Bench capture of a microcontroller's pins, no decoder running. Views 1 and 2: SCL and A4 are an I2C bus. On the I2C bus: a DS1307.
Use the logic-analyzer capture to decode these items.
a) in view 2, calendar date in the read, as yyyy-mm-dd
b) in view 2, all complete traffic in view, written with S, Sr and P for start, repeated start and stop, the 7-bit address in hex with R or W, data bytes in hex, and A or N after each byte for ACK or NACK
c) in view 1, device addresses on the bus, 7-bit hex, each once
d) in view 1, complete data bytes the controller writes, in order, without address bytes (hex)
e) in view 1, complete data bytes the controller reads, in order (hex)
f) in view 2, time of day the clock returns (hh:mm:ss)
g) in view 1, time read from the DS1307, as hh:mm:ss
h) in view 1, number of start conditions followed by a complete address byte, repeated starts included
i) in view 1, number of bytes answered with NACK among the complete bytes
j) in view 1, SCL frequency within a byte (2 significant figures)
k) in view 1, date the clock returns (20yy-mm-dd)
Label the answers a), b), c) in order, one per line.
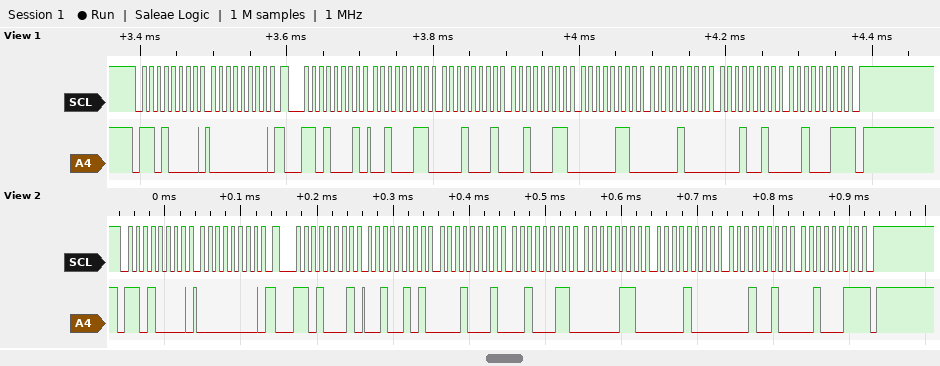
a) 2023-12-08
b) S 68W A 00 A Sr 68R A 25 A 11 A 23 A 06 A 08 A 12 A 23 N P
c) 0x68
d) 00
e) 23 11 23 06 08 12 23
f) 23:11:25
g) 23:11:23
h) 2
i) 1
j) 100 kHz
k) 2023-12-08
